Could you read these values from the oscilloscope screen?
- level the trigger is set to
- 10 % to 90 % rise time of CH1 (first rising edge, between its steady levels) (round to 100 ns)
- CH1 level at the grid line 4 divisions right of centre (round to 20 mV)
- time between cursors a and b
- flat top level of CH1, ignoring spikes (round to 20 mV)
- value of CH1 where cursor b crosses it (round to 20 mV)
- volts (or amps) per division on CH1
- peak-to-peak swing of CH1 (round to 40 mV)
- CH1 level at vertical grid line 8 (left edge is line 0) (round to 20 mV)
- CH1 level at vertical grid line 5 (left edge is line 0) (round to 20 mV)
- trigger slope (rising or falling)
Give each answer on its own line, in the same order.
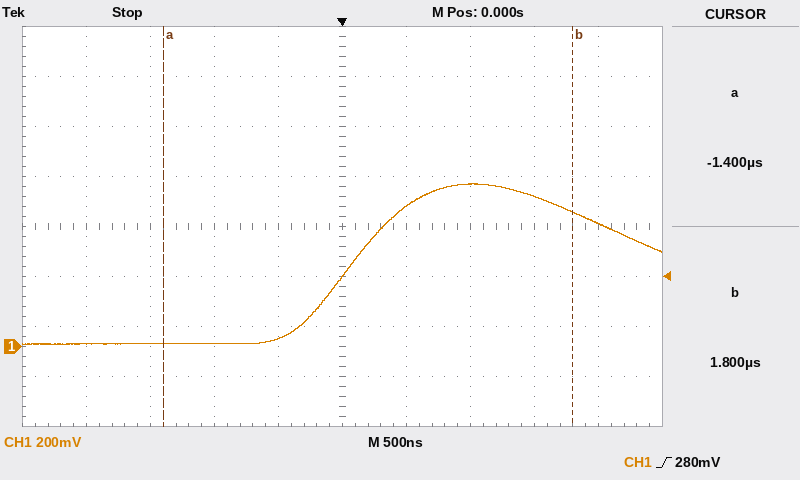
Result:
280 mV
900 ns
500 mV
3.20 µs
640 mV
540 mV
200 mV
640 mV
600 mV
280 mV
rising
